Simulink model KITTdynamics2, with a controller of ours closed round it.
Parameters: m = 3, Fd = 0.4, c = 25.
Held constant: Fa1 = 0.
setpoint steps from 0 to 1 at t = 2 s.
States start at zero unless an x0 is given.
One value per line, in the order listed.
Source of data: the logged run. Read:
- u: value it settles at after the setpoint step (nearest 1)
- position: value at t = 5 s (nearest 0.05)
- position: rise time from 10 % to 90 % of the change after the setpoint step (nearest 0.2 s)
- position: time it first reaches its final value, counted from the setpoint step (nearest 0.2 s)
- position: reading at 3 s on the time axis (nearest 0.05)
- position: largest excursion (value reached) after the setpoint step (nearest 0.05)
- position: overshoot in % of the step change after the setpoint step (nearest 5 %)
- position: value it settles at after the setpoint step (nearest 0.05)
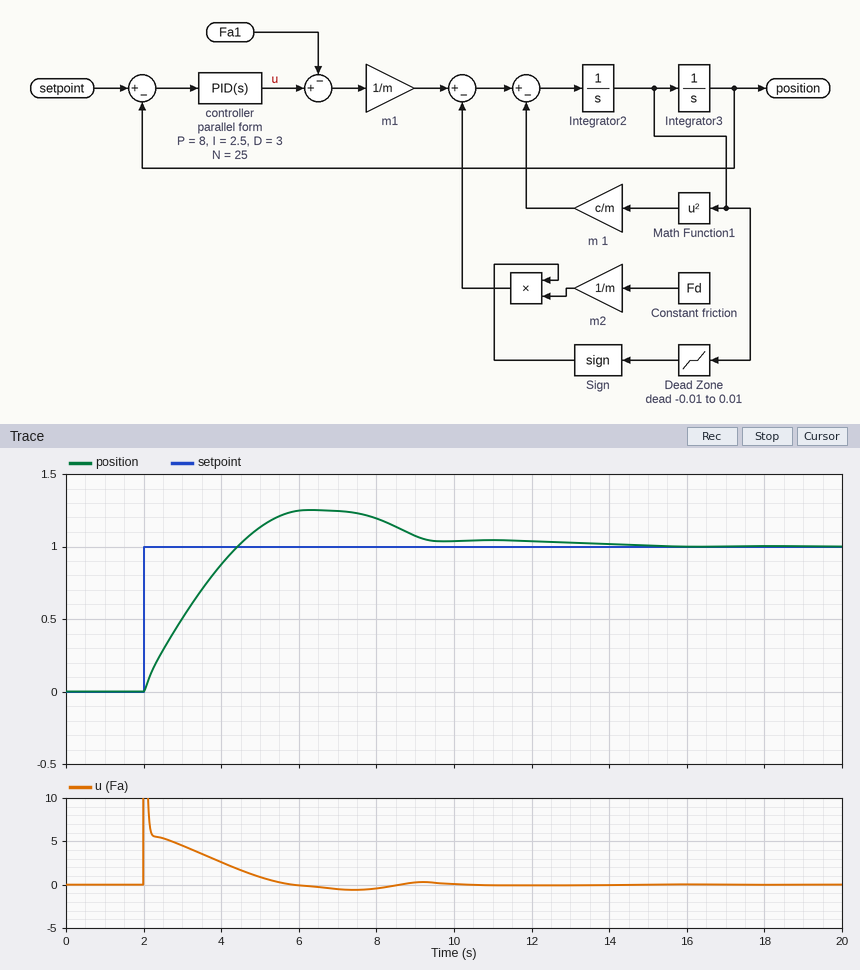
0
1.15
2.0 s
2.4 s
0.50
1.25
25 %
1.00
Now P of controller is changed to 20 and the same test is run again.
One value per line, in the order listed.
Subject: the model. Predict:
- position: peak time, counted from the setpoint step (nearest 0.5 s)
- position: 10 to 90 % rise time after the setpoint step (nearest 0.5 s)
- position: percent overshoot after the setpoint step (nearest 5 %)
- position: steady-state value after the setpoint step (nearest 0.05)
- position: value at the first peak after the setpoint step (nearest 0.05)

2.5 s
1.5 s
10 %
1.00
1.10
